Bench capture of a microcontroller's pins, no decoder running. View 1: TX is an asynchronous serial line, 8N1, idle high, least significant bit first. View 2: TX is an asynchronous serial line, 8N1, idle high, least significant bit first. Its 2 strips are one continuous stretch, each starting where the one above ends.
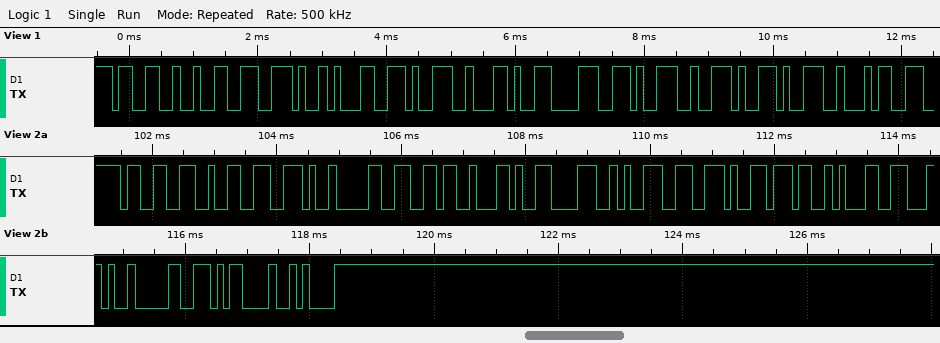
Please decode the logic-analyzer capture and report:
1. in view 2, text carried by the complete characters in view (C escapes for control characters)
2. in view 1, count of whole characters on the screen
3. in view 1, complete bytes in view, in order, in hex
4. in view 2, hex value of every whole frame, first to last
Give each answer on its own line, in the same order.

"32.06,89.71,0\r\n"
11
33 32 2E 31 39 2C 38 39 2E 39 34
33 32 2E 30 36 2C 38 39 2E 37 31 2C 30 0D 0A
